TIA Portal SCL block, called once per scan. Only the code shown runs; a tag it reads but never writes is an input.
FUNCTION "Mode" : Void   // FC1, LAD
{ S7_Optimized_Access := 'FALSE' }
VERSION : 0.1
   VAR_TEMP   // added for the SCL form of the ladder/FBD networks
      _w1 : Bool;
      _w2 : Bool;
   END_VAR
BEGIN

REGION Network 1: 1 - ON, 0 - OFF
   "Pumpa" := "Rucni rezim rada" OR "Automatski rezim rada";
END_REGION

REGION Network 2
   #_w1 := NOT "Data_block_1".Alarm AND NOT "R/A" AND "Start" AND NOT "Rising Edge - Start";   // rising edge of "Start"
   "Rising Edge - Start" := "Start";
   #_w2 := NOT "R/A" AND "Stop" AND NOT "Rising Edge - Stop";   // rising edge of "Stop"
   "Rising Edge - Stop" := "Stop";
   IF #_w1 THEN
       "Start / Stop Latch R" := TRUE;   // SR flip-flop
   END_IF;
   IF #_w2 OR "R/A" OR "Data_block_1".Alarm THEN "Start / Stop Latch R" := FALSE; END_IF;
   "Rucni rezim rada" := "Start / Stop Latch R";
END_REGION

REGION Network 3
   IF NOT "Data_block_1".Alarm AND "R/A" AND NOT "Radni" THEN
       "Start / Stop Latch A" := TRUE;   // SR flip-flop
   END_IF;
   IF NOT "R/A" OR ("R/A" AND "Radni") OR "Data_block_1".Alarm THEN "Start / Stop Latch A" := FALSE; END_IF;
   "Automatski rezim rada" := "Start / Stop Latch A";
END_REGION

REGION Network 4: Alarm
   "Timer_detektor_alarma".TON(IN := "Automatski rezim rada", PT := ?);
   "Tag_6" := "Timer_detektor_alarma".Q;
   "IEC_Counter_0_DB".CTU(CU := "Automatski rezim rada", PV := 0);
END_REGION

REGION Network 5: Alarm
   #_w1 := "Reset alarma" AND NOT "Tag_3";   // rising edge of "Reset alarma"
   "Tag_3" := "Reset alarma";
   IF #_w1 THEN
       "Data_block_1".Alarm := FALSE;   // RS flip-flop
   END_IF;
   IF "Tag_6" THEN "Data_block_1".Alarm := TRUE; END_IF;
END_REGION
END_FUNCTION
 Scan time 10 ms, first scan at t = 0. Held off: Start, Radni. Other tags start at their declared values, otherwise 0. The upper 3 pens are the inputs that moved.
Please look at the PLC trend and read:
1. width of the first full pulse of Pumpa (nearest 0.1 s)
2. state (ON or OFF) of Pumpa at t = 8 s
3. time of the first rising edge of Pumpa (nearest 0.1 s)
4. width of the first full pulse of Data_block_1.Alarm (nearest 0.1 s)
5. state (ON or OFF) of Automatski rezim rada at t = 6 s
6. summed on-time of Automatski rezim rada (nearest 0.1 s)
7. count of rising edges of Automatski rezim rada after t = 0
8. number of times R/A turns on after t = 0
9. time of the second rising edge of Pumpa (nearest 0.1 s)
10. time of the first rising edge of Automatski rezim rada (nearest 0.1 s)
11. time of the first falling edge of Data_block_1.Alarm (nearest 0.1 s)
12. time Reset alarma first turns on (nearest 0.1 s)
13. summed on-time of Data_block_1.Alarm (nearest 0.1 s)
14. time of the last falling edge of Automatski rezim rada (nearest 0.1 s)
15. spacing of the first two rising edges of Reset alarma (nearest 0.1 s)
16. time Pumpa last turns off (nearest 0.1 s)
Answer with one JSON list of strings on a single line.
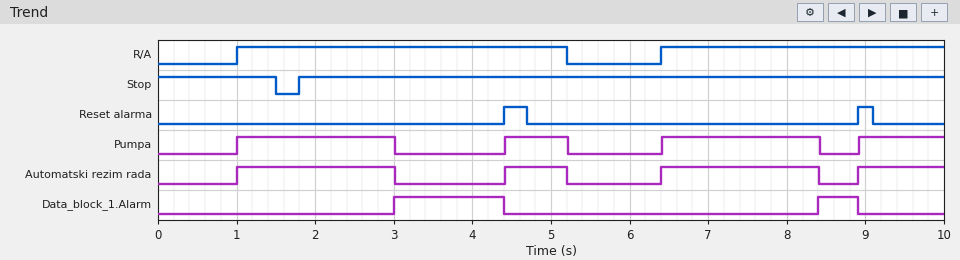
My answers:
["2.0 s", "ON", "1.0 s", "1.4 s", "OFF", "5.9 s", "4", "2", "4.4 s", "1.0 s", "4.4 s", "4.4 s", "1.9 s", "8.4 s", "4.5 s", "8.4 s"]
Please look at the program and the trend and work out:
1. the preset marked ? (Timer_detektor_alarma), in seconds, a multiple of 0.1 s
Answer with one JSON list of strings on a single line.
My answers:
["2.0 s"]
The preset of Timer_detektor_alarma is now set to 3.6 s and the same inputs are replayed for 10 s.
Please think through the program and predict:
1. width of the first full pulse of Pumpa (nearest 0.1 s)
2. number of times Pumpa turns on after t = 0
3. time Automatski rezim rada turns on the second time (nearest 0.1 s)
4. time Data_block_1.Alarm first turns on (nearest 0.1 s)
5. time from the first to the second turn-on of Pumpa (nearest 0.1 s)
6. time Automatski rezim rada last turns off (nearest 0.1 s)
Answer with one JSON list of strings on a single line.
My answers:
["3.6 s", "2", "8.9 s", "4.6 s", "7.9 s", "4.6 s"]
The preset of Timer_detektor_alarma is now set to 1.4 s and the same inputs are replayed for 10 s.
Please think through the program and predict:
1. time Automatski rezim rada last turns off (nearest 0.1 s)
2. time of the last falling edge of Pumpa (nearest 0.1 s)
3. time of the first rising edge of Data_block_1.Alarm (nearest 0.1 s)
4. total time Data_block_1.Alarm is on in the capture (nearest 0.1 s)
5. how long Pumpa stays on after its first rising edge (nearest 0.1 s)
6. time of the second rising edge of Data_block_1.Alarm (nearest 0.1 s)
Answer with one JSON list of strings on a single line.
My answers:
["7.8 s", "7.8 s", "2.4 s", "3.1 s", "1.4 s", "7.8 s"]
